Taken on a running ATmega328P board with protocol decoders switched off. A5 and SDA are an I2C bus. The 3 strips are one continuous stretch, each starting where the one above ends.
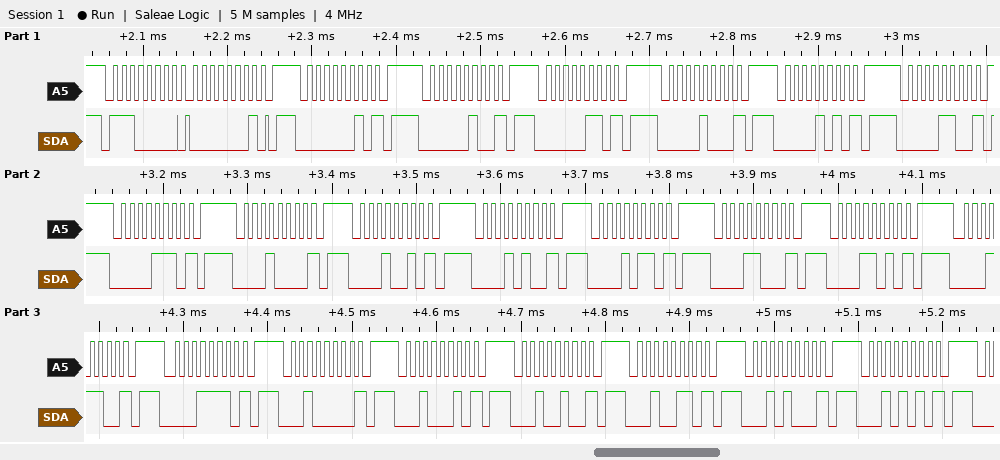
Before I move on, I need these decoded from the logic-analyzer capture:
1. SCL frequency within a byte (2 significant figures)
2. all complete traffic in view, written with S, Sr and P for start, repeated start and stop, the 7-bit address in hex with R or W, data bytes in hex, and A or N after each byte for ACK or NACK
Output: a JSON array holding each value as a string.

["100 kHz", "S 70W A 01 A P S 01W N P S 02W N P S 03W N P S 04W N P S 05W N P S 06W N P S 07W N P S 08W N P S 09W N P S 0AW N P S 0BW N P S 0CW N P S 0DW N P S 0EW N P S 0FW N P S 10W N P S 11W N P S 12W N P S 13W N P S 14W N P S 15W N P"]
